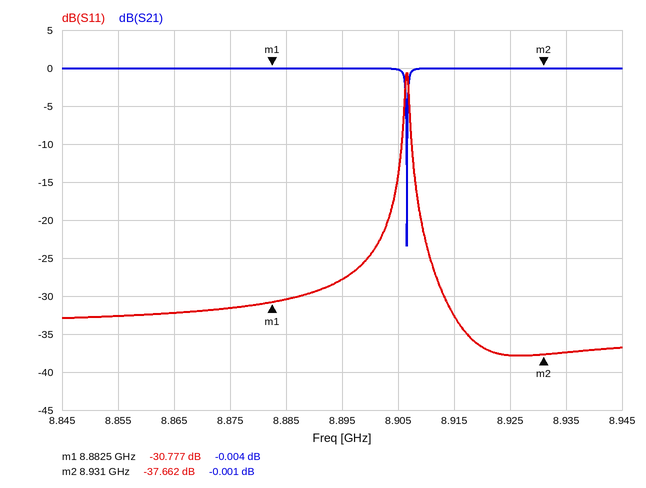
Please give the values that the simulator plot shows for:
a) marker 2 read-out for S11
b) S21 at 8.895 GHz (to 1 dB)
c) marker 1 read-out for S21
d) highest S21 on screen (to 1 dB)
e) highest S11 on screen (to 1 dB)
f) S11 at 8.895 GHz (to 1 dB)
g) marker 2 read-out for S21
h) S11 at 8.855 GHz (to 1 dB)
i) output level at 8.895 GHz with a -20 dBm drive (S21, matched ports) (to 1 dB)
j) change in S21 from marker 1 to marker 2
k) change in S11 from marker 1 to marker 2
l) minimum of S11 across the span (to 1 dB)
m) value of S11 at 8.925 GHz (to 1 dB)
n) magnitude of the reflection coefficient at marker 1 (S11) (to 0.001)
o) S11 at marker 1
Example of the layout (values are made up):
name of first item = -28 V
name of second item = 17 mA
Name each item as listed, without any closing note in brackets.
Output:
marker 2 read-out for S11 = -37.662 dB
S21 at 8.895 GHz = 0 dB
marker 1 read-out for S21 = -0.004 dB
highest S21 on screen = 0 dB
highest S11 on screen = -1 dB
S11 at 8.895 GHz = -28 dB
marker 2 read-out for S21 = -0.001 dB
S11 at 8.855 GHz = -33 dB
output level at 8.895 GHz with a -20 dBm drive (S21, matched ports) = -20 dBm
change in S21 from marker 1 to marker 2 = 0.003 dB
change in S11 from marker 1 to marker 2 = -6.885 dB
minimum of S11 across the span = -38 dB
value of S11 at 8.925 GHz = -38 dB
magnitude of the reflection coefficient at marker 1 (S11) = 0.029
S11 at marker 1 = -30.777 dB
